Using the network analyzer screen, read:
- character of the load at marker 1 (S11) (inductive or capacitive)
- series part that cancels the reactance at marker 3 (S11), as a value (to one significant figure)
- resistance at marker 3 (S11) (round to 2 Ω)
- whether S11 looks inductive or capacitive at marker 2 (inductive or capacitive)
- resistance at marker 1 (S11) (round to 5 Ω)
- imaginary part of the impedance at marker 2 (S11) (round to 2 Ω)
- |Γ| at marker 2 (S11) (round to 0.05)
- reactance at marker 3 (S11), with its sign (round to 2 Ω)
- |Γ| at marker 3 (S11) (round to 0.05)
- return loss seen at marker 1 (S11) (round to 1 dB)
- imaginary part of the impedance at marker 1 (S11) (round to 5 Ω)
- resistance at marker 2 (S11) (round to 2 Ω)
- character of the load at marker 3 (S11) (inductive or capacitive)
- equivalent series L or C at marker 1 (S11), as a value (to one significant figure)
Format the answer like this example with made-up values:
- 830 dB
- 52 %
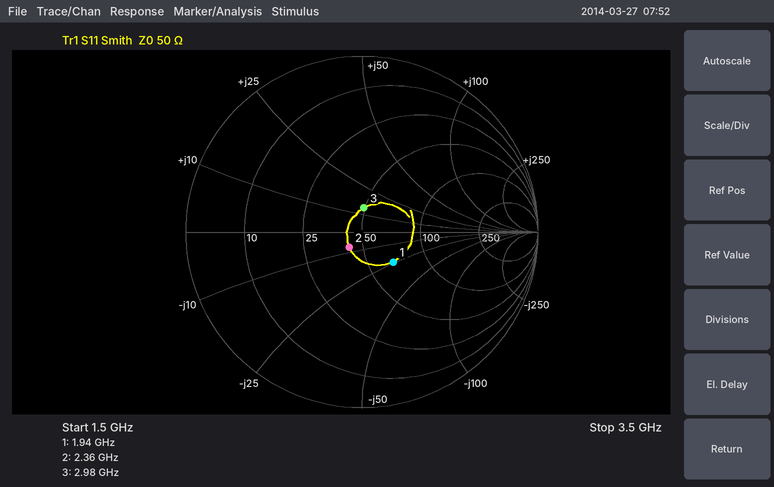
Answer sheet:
- capacitive
- 4 pF
- 50 Ω
- capacitive
- 65 Ω
- -8 Ω
- 0.10
- +14 Ω
- 0.15
- 12 dB
- -25 Ω
- 42 Ω
- inductive
- 3 pF
